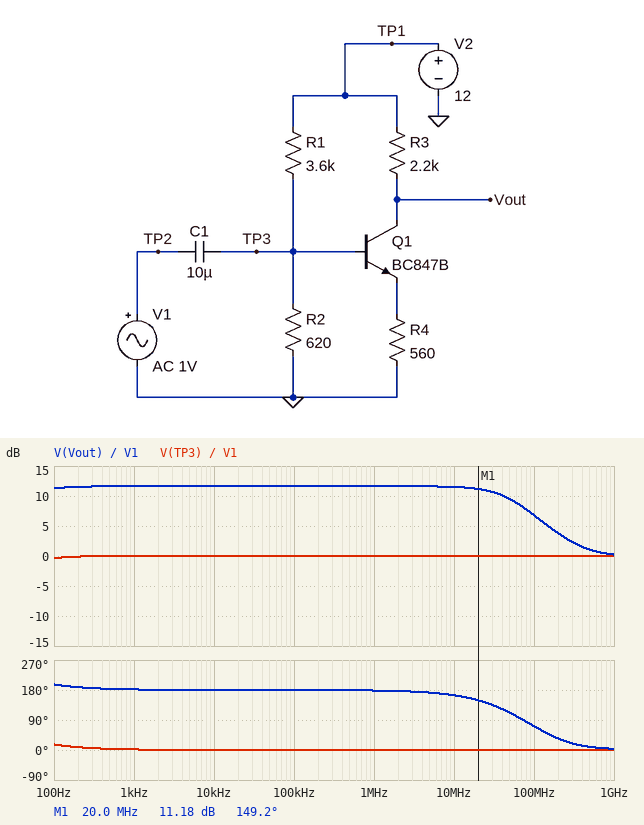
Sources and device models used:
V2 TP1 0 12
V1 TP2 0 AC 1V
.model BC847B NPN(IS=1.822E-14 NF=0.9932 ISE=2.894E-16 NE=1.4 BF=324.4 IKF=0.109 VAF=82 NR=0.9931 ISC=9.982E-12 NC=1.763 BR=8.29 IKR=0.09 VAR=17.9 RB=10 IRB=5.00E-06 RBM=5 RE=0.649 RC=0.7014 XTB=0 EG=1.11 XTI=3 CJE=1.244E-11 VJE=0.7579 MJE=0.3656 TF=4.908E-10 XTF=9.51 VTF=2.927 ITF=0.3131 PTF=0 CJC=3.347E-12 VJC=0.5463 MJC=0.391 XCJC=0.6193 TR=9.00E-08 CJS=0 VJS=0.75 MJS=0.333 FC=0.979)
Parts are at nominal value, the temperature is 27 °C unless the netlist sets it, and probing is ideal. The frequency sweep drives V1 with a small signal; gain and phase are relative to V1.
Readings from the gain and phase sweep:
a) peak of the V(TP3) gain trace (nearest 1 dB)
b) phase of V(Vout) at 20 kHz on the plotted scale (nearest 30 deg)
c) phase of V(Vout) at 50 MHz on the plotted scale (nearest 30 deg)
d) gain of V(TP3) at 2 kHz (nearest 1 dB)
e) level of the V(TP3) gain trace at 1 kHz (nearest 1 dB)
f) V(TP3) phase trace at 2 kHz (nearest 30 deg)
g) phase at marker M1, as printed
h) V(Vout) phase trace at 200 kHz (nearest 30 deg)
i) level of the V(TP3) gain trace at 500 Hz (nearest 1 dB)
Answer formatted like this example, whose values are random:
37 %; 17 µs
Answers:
0 dB; 180 deg; 120 deg; 0 dB; 0 dB; 0 deg; 149.2 deg; 180 deg; 0 dB
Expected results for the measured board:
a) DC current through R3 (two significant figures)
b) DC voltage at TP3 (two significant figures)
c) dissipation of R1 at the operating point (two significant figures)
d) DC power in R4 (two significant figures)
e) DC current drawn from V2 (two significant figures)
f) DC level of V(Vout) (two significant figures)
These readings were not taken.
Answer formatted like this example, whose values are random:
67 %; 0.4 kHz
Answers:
2.0 mA; 1.8 V; 29 mW; 2.2 mW; 4.8 mA; 7.7 V
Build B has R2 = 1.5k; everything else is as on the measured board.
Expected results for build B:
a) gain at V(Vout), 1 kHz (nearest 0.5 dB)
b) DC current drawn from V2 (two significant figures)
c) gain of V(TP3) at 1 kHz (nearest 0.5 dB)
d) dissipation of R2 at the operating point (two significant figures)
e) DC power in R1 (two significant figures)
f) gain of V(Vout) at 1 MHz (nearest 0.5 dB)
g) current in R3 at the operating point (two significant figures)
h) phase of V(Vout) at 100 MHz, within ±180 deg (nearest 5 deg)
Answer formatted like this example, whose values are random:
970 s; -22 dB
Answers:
-2.0 dB; 6.7 mA; 0 dB; 7.0 mW; 21 mW; 0 dB; 4.3 mA; 0 deg
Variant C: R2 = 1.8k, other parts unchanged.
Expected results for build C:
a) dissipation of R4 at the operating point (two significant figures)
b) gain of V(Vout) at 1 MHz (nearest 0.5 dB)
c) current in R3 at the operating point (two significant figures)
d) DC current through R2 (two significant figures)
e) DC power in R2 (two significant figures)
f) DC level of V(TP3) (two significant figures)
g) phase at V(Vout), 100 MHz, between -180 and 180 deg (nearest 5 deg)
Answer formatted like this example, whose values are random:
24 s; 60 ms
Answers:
13 mW; 0 dB; 4.2 mA; 1.9 mA; 6.3 mW; 3.4 V; 0 deg
